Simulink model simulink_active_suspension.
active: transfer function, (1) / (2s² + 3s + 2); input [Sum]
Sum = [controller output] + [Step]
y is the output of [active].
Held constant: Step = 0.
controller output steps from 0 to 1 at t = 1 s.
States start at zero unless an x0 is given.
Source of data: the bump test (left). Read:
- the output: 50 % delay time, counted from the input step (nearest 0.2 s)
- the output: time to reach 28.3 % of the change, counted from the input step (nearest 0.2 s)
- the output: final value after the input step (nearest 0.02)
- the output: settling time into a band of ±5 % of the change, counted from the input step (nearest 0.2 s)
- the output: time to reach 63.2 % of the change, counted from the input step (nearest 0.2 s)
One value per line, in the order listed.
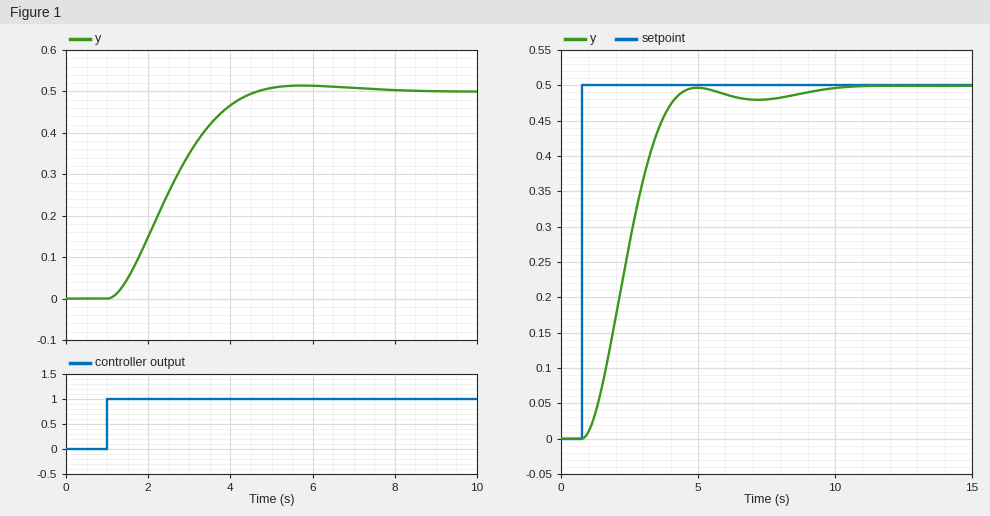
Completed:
1.4 s
1.0 s
0.50
3.2 s
1.8 s
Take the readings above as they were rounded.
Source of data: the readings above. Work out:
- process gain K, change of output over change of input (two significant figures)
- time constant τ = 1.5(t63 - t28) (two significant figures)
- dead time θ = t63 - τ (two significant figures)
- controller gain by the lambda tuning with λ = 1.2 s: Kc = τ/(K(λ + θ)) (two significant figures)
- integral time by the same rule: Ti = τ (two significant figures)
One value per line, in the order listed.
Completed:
0.50
1.2 s
0.60 s
1.3
1.2 s
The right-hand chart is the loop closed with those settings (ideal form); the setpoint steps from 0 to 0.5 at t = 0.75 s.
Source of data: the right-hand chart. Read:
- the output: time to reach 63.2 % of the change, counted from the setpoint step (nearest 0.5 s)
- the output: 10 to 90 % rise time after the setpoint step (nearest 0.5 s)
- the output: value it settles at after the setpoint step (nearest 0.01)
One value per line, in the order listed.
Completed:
2.0 s
2.5 s
0.50
